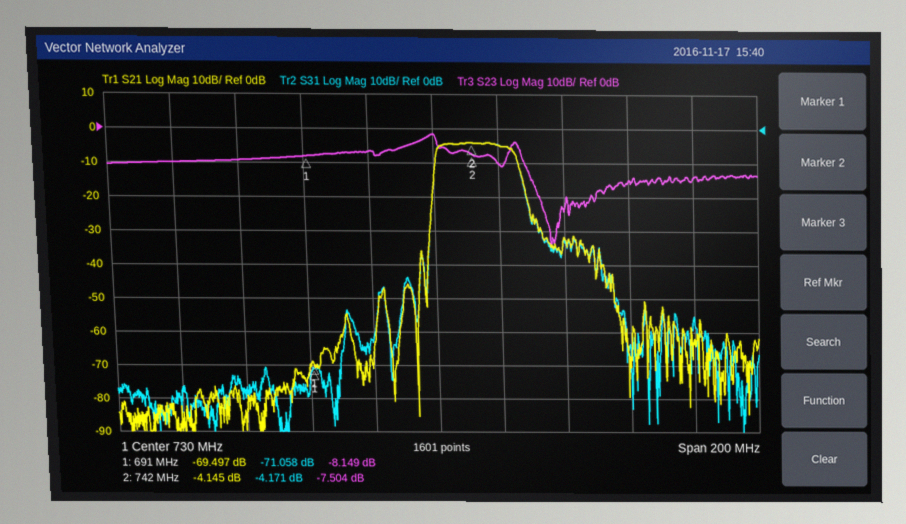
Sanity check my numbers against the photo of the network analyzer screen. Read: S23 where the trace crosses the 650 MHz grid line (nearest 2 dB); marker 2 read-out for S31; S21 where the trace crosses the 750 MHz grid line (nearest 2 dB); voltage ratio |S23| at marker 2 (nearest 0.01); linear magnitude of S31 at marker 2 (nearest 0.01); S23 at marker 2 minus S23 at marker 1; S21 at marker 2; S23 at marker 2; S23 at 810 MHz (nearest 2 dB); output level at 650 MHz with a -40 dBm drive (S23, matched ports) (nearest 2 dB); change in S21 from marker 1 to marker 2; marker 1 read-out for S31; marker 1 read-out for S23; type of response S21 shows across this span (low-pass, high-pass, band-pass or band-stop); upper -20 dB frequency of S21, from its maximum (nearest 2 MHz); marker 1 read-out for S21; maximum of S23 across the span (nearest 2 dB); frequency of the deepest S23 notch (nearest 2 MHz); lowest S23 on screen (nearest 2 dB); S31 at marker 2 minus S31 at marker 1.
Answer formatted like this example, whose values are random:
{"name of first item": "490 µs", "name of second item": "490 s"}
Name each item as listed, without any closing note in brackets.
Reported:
{"S23 where the trace crosses the 650 MHz grid line": "-10 dB", "marker 2 read-out for S31": "-4.171 dB", "S21 where the trace crosses the 750 MHz grid line": "-4 dB", "voltage ratio |S23| at marker 2": "0.42", "linear magnitude of S31 at marker 2": "0.62", "S23 at marker 2 minus S23 at marker 1": "0.645 dB", "S21 at marker 2": "-4.145 dB", "S23 at marker 2": "-7.504 dB", "S23 at 810 MHz": "-14 dB", "output level at 650 MHz with a -40 dBm drive (S23, matched ports)": "-50 dBm", "change in S21 from marker 1 to marker 2": "65.352 dB", "marker 1 read-out for S31": "-71.058 dB", "marker 1 read-out for S23": "-8.149 dB", "type of response S21 shows across this span": "band-pass", "upper -20 dB frequency of S21, from its maximum": "760 MHz", "marker 1 read-out for S21": "-69.497 dB", "maximum of S23 across the span": "-2 dB", "frequency of the deepest S23 notch": "766 MHz", "lowest S23 on screen": "-34 dB", "S31 at marker 2 minus S31 at marker 1": "66.887 dB"}
